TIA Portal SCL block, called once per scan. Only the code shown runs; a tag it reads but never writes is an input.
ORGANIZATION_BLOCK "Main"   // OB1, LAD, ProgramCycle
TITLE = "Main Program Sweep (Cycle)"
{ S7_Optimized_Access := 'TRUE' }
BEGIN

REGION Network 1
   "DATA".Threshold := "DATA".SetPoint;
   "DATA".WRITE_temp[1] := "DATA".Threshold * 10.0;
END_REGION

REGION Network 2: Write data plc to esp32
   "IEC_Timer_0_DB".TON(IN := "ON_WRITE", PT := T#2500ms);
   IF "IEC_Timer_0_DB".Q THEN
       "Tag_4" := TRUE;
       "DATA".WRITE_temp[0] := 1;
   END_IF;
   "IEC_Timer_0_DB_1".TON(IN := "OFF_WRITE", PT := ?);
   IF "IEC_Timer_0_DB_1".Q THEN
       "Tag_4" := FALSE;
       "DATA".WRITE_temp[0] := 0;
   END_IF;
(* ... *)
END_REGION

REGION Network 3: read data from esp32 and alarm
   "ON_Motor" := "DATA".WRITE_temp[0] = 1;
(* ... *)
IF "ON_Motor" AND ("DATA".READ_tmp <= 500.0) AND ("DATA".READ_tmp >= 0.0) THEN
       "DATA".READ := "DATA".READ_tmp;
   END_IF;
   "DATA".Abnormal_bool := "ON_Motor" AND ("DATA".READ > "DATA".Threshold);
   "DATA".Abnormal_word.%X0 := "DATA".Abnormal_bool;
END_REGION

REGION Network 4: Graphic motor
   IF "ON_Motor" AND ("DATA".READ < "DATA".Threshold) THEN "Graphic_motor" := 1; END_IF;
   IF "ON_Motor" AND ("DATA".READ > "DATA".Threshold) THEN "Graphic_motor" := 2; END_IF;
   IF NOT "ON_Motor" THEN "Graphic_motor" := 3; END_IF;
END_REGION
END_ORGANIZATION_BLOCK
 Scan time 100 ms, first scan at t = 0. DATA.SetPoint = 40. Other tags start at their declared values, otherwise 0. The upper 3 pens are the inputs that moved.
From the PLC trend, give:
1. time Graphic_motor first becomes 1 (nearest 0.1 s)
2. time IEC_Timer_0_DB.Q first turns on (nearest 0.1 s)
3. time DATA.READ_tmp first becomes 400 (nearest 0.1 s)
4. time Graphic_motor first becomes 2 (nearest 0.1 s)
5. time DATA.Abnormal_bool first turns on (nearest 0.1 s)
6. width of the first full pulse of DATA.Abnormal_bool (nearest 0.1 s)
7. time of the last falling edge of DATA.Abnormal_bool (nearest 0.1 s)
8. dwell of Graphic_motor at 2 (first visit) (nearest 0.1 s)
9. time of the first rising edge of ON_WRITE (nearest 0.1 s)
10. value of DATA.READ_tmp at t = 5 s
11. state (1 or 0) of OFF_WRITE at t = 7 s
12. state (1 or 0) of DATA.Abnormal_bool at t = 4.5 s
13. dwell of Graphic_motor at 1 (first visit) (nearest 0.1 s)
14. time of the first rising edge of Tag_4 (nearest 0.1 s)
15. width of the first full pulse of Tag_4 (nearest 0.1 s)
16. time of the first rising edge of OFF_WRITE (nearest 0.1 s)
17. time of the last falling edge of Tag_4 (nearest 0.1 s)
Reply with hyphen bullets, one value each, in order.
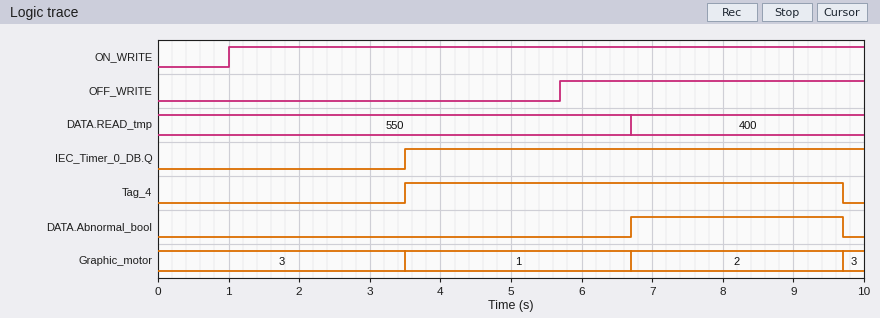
- 3.5 s
- 3.5 s
- 6.7 s
- 6.7 s
- 6.7 s
- 3.0 s
- 9.7 s
- 3.0 s
- 1.0 s
- 550
- 1
- 0
- 3.2 s
- 3.5 s
- 6.2 s
- 5.7 s
- 9.7 s
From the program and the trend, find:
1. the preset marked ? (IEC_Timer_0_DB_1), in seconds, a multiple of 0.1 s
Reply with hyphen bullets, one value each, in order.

- 4.0 s
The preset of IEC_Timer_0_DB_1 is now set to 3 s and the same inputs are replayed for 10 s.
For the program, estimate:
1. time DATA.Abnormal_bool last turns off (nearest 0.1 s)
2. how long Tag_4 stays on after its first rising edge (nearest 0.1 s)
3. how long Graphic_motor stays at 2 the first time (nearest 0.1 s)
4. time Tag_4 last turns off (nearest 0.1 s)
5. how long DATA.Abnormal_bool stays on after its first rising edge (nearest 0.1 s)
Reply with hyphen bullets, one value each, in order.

- 8.7 s
- 5.2 s
- 2.0 s
- 8.7 s
- 2.0 s
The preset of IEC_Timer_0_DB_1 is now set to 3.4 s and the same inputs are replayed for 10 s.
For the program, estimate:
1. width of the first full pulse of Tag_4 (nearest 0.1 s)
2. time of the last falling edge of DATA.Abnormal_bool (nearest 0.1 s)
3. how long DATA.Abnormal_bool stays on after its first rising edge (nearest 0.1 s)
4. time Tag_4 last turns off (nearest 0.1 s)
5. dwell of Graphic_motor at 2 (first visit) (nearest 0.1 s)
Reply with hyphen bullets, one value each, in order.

- 5.6 s
- 9.1 s
- 2.4 s
- 9.1 s
- 2.4 s
